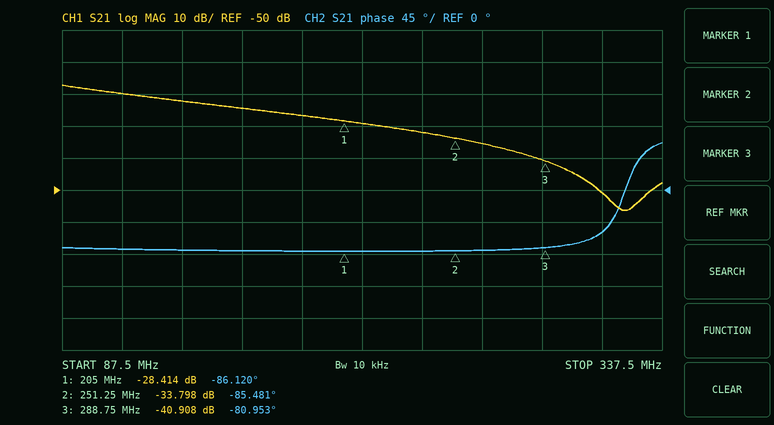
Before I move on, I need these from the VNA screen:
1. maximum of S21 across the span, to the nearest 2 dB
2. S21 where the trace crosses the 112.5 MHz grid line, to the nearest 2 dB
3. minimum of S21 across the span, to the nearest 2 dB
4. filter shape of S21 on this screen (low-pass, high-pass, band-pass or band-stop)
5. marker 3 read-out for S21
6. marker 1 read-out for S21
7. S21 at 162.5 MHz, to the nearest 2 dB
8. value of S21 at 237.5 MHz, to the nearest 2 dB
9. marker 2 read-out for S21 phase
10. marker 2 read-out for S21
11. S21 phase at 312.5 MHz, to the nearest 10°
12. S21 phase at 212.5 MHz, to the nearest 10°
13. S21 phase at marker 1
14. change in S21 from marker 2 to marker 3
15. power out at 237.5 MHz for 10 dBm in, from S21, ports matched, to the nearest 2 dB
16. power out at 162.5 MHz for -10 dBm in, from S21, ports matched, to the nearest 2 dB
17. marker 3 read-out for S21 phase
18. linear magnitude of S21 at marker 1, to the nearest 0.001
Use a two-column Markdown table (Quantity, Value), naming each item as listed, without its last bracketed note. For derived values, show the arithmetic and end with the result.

| Quantity | Value |
|---|---|
| maximum of S21 across the span, to the nearest 2 dB | -18 dB |
| S21 where the trace crosses the 112.5 MHz grid line, to the nearest 2 dB | -20 dB |
| minimum of S21 across the span, to the nearest 2 dB | -56 dB |
| filter shape of S21 on this screen | low-pass |
| marker 3 read-out for S21 | -40.908 dB |
| marker 1 read-out for S21 | -28.414 dB |
| S21 at 162.5 MHz, to the nearest 2 dB | -24 dB |
| value of S21 at 237.5 MHz, to the nearest 2 dB | -32 dB |
| marker 2 read-out for S21 phase | -85.481° |
| marker 2 read-out for S21 | -33.798 dB |
| S21 phase at 312.5 MHz, to the nearest 10° | -60° |
| S21 phase at 212.5 MHz, to the nearest 10° | -90° |
| S21 phase at marker 1 | -86.120° |
| change in S21 from marker 2 to marker 3 | -40.908 − (-33.798) = -7.110 dB |
| power out at 237.5 MHz for 10 dBm in, from S21, ports matched, to the nearest 2 dB | 10 dBm + (-32 dB) = -22 dBm |
| power out at 162.5 MHz for -10 dBm in, from S21, ports matched, to the nearest 2 dB | -10 dBm + (-24 dB) = -34 dBm |
| marker 3 read-out for S21 phase | -80.953° |
| linear magnitude of S21 at marker 1, to the nearest 0.001 | 10^(-28.414/20) ≈ 0.038 |
